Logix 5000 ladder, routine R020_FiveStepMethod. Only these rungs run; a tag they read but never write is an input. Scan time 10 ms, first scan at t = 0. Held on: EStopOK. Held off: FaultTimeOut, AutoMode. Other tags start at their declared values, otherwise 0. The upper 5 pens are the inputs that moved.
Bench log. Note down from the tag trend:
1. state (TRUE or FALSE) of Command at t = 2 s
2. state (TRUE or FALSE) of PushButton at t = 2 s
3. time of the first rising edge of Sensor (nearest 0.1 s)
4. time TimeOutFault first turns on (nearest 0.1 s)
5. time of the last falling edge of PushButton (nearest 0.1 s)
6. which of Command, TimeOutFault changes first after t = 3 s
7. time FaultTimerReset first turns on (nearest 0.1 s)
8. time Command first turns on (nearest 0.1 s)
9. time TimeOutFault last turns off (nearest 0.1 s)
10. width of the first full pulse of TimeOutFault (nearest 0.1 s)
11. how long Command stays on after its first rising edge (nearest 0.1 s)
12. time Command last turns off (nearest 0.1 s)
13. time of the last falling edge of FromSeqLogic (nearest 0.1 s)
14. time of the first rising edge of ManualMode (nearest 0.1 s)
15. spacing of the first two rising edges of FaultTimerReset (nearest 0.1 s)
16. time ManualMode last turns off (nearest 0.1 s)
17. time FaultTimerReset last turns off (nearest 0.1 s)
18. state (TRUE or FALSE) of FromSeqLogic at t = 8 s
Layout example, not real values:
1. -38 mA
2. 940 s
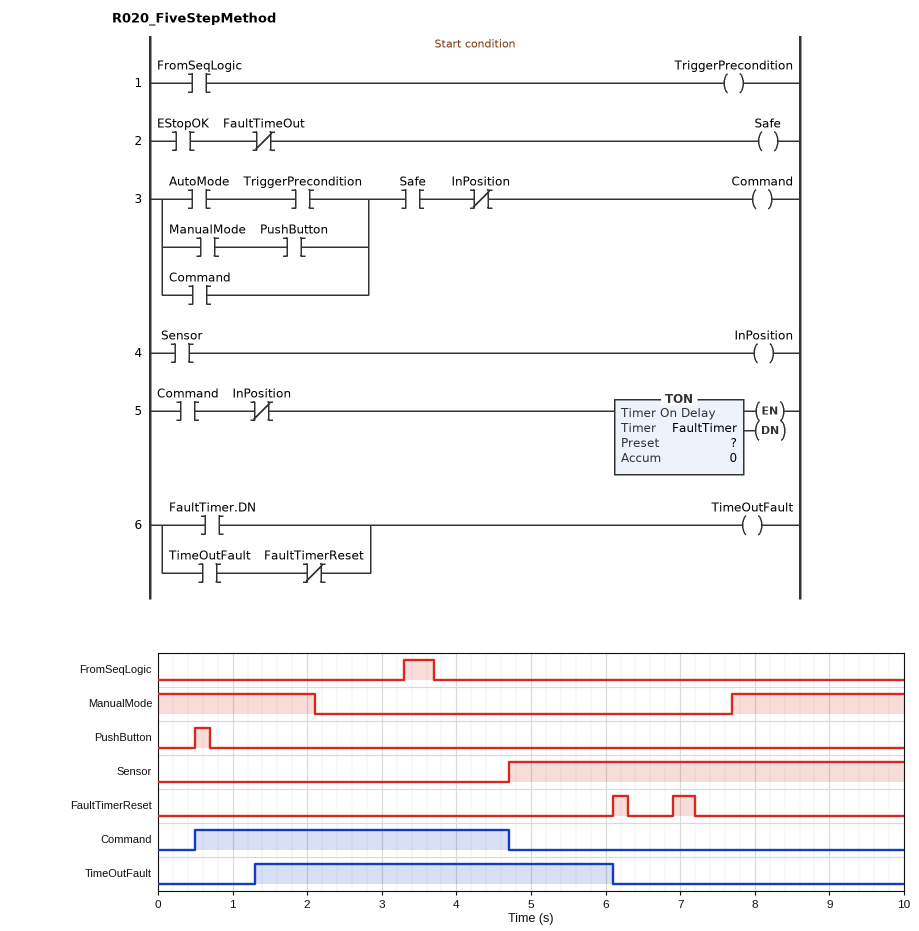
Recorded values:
1. TRUE
2. FALSE
3. 4.7 s
4. 1.3 s
5. 0.7 s
6. Command
7. 6.1 s
8. 0.5 s
9. 6.1 s
10. 4.8 s
11. 4.2 s
12. 4.7 s
13. 3.7 s
14. 7.7 s
15. 0.8 s
16. 2.1 s
17. 7.2 s
18. FALSE
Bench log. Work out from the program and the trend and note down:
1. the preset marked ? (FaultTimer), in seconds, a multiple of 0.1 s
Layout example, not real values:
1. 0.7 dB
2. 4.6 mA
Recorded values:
1. 0.8 s
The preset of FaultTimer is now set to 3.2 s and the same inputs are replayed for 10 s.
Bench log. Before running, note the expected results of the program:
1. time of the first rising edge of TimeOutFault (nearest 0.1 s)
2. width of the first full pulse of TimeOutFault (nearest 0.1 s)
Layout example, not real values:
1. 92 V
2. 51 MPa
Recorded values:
1. 3.7 s
2. 2.4 s
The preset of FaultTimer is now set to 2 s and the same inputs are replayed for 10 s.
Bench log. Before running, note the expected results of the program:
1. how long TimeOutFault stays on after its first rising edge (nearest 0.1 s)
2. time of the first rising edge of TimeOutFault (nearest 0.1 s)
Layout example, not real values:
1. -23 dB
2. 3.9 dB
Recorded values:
1. 3.6 s
2. 2.5 s
